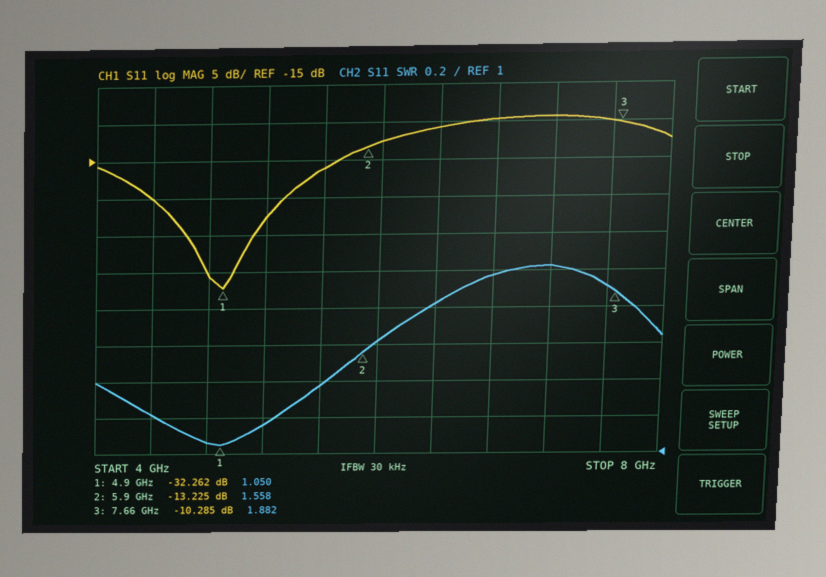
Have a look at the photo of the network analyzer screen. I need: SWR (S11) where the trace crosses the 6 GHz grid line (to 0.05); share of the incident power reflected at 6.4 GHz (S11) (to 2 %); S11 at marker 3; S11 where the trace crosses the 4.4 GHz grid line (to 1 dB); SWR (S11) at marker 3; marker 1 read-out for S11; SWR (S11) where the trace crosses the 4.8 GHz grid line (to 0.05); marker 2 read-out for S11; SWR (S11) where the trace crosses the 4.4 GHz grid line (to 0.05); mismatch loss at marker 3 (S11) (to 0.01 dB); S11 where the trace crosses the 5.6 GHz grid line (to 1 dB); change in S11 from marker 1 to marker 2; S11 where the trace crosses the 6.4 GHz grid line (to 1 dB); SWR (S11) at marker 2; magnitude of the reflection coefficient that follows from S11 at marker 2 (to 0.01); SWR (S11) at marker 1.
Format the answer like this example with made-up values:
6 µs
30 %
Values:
1.60
8 %
-10.285 dB
-20 dB
1.882
-32.262 dB
1.05
-13.225 dB
1.20
0.43 dB
-16 dB
19.037 dB
-11 dB
1.558
0.22
1.050
